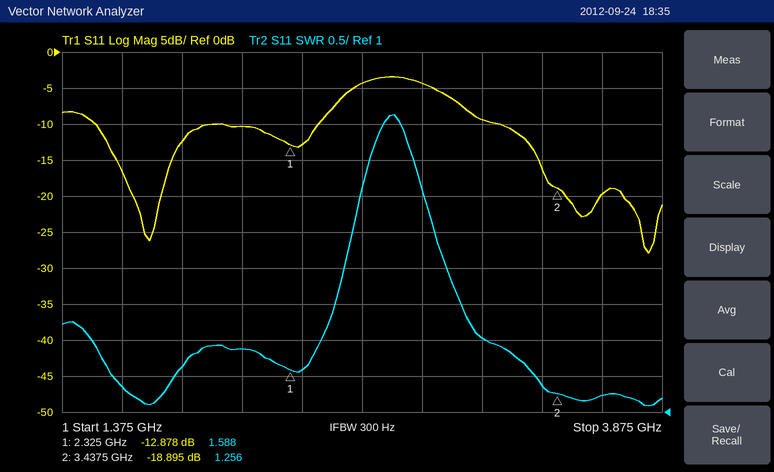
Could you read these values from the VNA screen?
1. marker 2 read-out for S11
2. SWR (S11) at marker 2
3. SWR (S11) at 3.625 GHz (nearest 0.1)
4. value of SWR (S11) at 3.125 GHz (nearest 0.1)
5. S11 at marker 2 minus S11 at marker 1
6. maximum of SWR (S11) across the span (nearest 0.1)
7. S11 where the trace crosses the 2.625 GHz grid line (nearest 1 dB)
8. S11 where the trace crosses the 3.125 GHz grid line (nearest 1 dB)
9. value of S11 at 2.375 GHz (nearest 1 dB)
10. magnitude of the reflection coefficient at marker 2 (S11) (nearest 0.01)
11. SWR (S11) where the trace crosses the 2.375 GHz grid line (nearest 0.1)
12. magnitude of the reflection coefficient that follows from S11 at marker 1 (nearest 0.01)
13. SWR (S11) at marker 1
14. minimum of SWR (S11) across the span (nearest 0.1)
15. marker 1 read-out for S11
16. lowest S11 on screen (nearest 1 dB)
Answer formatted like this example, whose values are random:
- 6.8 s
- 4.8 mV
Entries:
- -18.895 dB
- 1.256
- 1.2
- 2.0
- -6.017 dB
- 5.1
- -4 dB
- -9 dB
- -13 dB
- 0.11
- 1.6
- 0.23
- 1.588
- 1.1
- -12.878 dB
- -28 dB
